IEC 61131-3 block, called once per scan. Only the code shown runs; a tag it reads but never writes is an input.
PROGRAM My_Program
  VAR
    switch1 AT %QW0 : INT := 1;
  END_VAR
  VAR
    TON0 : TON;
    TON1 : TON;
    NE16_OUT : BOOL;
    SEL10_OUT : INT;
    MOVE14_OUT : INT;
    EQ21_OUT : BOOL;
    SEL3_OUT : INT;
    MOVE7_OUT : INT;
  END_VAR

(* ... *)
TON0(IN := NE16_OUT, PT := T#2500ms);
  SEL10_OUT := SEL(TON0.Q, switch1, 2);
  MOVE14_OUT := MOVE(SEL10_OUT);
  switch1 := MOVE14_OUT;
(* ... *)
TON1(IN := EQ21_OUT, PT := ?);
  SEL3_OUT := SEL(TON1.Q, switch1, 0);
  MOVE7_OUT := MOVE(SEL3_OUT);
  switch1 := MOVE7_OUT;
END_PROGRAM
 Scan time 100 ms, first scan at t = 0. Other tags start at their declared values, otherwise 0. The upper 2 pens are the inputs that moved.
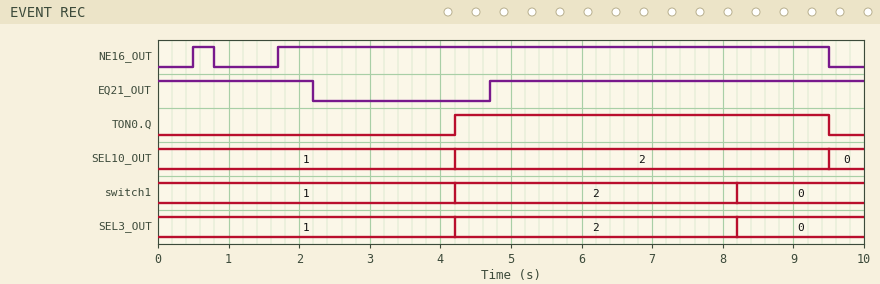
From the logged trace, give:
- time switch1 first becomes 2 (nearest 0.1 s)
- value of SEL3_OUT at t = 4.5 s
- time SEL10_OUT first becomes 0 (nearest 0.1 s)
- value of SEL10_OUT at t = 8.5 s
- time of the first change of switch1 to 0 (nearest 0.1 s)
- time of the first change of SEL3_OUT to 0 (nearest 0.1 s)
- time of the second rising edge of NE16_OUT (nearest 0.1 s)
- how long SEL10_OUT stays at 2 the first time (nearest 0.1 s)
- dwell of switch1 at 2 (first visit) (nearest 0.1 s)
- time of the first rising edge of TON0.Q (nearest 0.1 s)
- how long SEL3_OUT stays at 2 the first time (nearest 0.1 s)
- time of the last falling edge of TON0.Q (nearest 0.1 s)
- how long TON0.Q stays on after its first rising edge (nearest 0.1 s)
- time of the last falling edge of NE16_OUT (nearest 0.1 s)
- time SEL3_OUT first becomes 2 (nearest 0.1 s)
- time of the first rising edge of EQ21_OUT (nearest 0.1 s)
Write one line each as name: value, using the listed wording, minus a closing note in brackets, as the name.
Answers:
time switch1 first becomes 2: 4.2 s
value of SEL3_OUT at t = 4.5 s: 2
time SEL10_OUT first becomes 0: 9.5 s
value of SEL10_OUT at t = 8.5 s: 2
time of the first change of switch1 to 0: 8.2 s
time of the first change of SEL3_OUT to 0: 8.2 s
time of the second rising edge of NE16_OUT: 1.7 s
how long SEL10_OUT stays at 2 the first time: 5.3 s
dwell of switch1 at 2 (first visit): 4.0 s
time of the first rising edge of TON0.Q: 4.2 s
how long SEL3_OUT stays at 2 the first time: 4.0 s
time of the last falling edge of TON0.Q: 9.5 s
how long TON0.Q stays on after its first rising edge: 5.3 s
time of the last falling edge of NE16_OUT: 9.5 s
time SEL3_OUT first becomes 2: 4.2 s
time of the first rising edge of EQ21_OUT: 4.7 s
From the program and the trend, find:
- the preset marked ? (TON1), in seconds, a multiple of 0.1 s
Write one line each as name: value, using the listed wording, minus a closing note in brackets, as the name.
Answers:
the preset marked ? (TON1), in seconds, a multiple of 0.1 s: 3.5 s
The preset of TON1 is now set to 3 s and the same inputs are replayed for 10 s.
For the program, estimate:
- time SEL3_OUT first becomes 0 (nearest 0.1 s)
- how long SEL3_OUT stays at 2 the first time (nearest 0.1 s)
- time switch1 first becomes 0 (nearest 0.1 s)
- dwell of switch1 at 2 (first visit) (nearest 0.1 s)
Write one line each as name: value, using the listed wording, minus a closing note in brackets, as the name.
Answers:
time SEL3_OUT first becomes 0: 7.7 s
how long SEL3_OUT stays at 2 the first time: 3.5 s
time switch1 first becomes 0: 7.7 s
dwell of switch1 at 2 (first visit): 3.5 s
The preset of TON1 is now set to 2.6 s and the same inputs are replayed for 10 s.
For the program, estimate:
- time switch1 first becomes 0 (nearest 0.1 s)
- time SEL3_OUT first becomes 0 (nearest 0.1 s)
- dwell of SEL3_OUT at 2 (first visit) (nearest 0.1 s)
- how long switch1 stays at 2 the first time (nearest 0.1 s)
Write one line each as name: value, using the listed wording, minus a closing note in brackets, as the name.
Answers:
time switch1 first becomes 0: 7.3 s
time SEL3_OUT first becomes 0: 7.3 s
dwell of SEL3_OUT at 2 (first visit): 3.1 s
how long switch1 stays at 2 the first time: 3.1 s
